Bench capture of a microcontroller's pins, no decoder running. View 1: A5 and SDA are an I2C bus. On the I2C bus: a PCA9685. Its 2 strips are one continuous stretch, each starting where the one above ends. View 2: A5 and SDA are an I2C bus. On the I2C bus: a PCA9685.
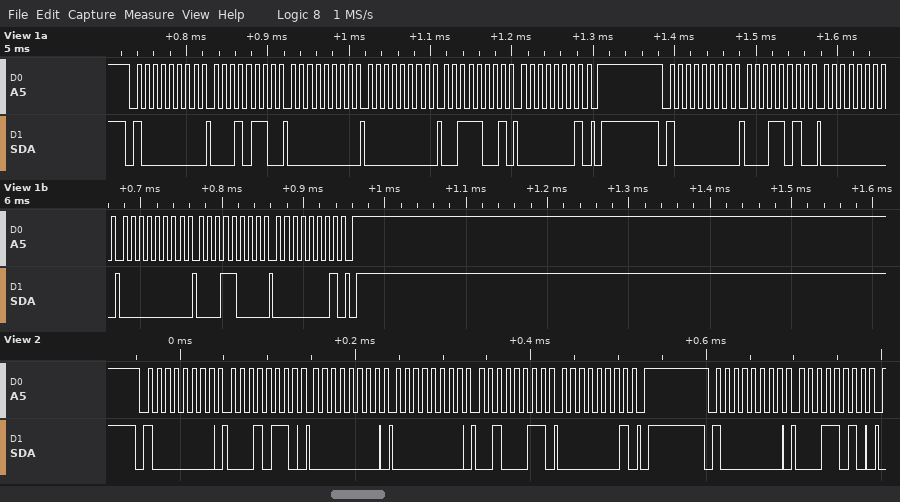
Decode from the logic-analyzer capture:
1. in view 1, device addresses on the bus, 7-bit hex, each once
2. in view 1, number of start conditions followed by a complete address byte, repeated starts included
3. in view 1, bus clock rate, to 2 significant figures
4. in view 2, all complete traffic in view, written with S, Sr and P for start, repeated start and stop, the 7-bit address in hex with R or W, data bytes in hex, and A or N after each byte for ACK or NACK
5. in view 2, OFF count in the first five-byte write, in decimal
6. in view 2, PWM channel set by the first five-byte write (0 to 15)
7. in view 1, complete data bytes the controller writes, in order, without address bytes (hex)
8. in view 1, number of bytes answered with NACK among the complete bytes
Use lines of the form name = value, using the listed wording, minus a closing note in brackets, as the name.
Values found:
in view 1, device addresses on the bus, 7-bit hex, each once = 0x40
in view 1, number of start conditions followed by a complete address byte, repeated starts included = 2
in view 1, bus clock rate, to 2 significant figures = 100 kHz
in view 2, all complete traffic in view, written with S, Sr and P for start, repeated start and stop, the 7-bit address in hex with R or W, data bytes in hex, and A or N after each byte for ACK or NACK = S 40W A 16 A 00 A 00 A 23 A 01 A P S 40W A 1A A
in view 2, OFF count in the first five-byte write, in decimal = 291
in view 2, PWM channel set by the first five-byte write = 4
in view 1, complete data bytes the controller writes, in order, without address bytes = 16 00 00 39 01 1A 00 00 18 01
in view 1, number of bytes answered with NACK among the complete bytes = 0
